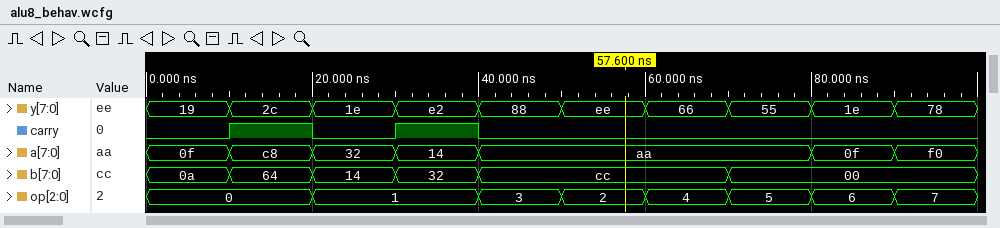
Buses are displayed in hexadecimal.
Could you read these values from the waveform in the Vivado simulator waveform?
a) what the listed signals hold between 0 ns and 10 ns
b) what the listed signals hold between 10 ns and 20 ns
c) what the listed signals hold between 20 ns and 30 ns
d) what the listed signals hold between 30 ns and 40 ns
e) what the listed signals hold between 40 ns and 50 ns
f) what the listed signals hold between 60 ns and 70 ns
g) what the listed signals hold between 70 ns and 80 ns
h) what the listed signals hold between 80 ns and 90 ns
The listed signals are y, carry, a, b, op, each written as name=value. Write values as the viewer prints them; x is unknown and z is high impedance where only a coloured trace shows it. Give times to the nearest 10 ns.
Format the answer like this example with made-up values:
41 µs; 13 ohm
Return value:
y=19, carry=0, a=0f, b=0a, op=0; y=2c, carry=1, a=c8, b=64, op=0; y=1e, carry=0, a=32, b=14, op=1; y=e2, carry=1, a=14, b=32, op=1; y=88, carry=0, a=aa, b=cc, op=3; y=66, carry=0, a=aa, b=cc, op=4; y=55, carry=0, a=aa, b=00, op=5; y=1e, carry=0, a=0f, b=00, op=6
